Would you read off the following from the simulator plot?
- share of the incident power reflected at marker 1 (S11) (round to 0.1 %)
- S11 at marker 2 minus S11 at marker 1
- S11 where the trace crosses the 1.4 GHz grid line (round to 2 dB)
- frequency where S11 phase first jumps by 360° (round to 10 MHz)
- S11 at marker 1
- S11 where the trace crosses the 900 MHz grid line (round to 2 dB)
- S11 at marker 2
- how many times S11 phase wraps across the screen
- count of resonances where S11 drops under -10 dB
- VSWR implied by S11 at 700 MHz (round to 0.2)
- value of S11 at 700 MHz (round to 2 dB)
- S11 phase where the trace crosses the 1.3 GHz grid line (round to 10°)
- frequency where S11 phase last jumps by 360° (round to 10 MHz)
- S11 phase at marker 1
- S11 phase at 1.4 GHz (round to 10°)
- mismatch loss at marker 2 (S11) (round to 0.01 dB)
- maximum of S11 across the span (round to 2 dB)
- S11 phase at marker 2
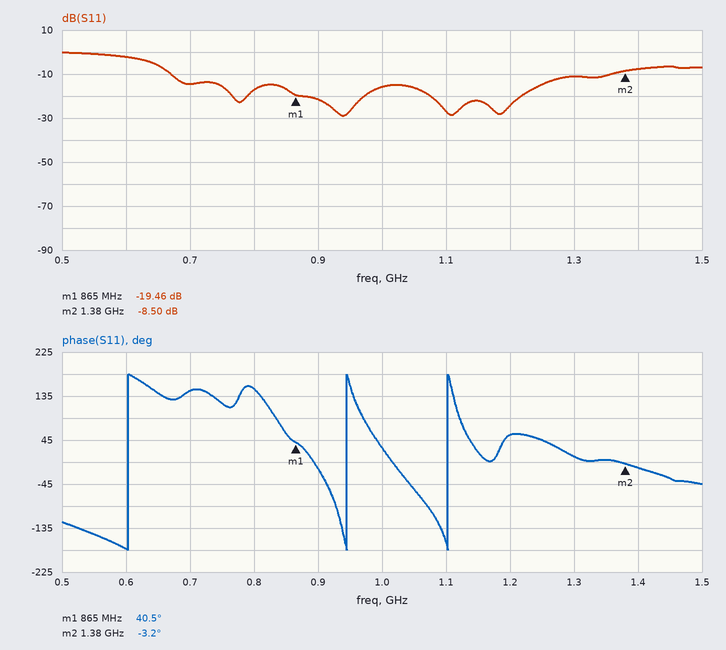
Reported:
1.1 %
10.96 dB
-8 dB
600 MHz
-19.46 dB
-22 dB
-8.50 dB
3
4
1.4
-14 dB
10°
1.10 GHz
40.5°
-10°
0.66 dB
0 dB
-3.2°
